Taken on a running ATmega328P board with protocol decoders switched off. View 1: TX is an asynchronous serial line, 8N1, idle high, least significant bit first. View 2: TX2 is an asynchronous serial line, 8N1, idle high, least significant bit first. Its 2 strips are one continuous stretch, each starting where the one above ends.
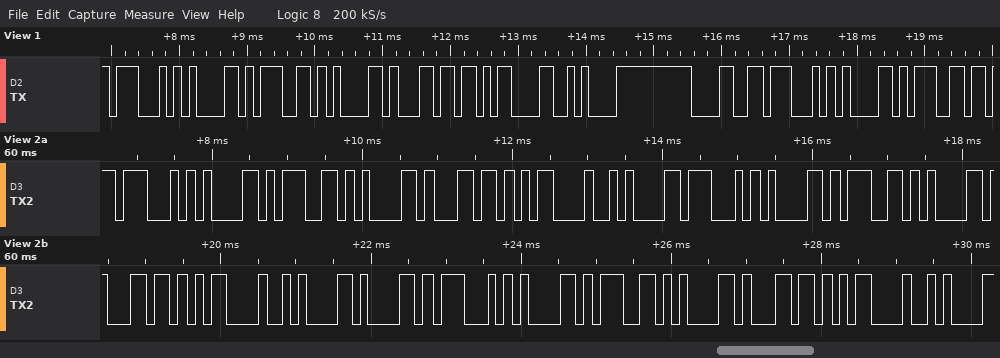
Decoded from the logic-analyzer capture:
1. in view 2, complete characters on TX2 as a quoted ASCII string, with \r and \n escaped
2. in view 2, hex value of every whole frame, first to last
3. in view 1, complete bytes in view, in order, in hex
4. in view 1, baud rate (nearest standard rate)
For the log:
"Gagal\r\nGagal\r\naGagal\r\n"
47 61 67 61 6C 0D 0A 47 61 67 61 6C 0D 0A 61 47 61 67 61 6C 0D 0A
47 61 67 61 6C 0D 0A 98 47 61 67
9600 baud
